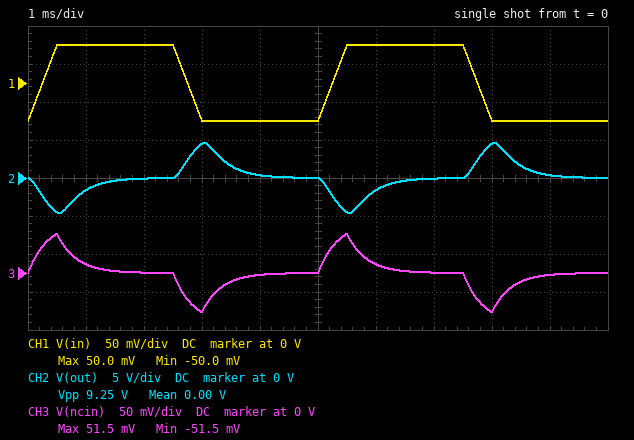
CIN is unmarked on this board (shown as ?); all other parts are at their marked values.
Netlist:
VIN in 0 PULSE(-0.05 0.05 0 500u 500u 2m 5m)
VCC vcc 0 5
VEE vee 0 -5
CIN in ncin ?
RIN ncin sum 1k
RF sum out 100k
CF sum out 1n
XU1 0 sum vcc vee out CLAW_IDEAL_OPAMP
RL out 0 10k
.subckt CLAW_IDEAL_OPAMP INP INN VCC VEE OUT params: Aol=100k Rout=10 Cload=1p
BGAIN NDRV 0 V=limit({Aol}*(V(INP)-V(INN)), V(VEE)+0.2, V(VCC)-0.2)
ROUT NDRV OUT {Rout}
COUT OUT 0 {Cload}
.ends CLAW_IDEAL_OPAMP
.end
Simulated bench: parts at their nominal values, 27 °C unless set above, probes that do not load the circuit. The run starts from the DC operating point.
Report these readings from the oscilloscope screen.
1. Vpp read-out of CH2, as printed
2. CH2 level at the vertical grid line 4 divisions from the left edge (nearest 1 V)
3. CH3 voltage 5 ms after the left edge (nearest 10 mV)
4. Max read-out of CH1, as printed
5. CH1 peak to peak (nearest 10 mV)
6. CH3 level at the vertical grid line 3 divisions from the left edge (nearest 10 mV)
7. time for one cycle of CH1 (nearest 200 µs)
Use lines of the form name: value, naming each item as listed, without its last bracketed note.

Vpp read-out of CH2, as printed: 9.25 V
CH2 level at the vertical grid line 4 divisions from the left edge: 0 V
CH3 voltage 5 ms after the left edge: 0 V
Max read-out of CH1, as printed: 50.0 mV
CH1 peak to peak: 100 mV
CH3 level at the vertical grid line 3 divisions from the left edge: -50 mV
time for one cycle of CH1: 5.0 ms
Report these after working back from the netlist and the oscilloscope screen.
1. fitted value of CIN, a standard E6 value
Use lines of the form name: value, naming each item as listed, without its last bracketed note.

fitted value of CIN, a standard E6 value: 330 nF
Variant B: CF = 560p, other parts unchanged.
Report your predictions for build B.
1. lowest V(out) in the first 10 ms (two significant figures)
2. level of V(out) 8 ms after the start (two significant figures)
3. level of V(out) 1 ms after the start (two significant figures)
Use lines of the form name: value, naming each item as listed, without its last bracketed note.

lowest V(out) in the first 10 ms: -4.8 V
level of V(out) 8 ms after the start: 4.8 V
level of V(out) 1 ms after the start: -1.4 V
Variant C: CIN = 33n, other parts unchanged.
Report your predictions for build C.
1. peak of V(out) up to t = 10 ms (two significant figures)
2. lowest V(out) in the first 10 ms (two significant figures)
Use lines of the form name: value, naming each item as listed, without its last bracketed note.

peak of V(out) up to t = 10 ms: 650 mV
lowest V(out) in the first 10 ms: -650 mV
